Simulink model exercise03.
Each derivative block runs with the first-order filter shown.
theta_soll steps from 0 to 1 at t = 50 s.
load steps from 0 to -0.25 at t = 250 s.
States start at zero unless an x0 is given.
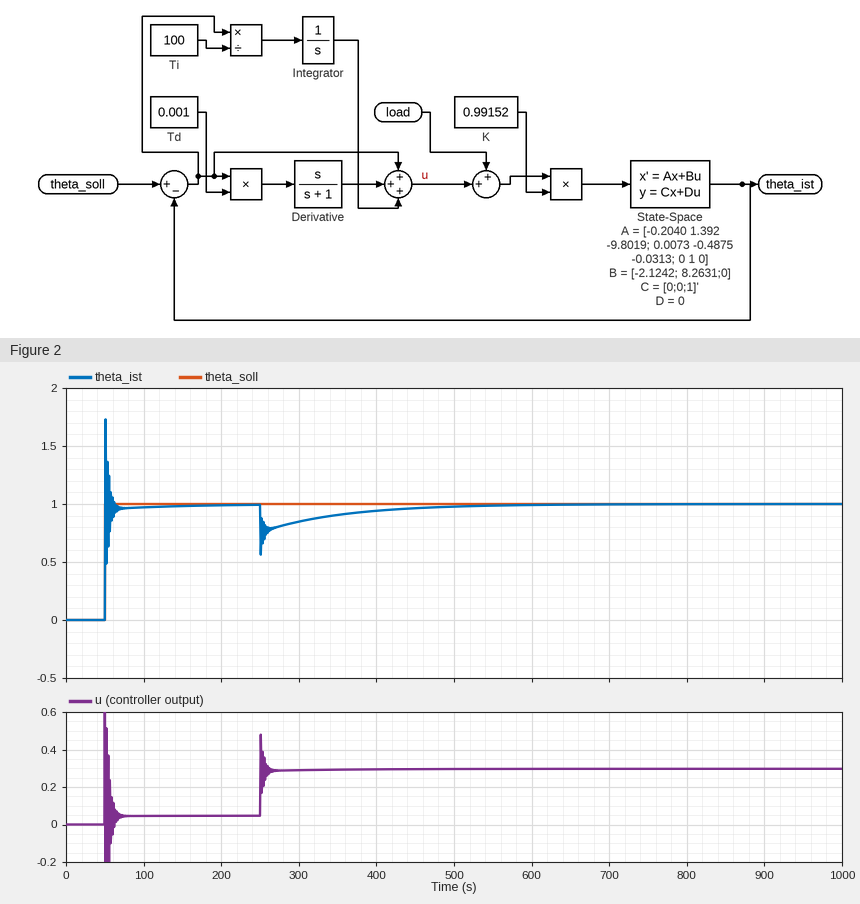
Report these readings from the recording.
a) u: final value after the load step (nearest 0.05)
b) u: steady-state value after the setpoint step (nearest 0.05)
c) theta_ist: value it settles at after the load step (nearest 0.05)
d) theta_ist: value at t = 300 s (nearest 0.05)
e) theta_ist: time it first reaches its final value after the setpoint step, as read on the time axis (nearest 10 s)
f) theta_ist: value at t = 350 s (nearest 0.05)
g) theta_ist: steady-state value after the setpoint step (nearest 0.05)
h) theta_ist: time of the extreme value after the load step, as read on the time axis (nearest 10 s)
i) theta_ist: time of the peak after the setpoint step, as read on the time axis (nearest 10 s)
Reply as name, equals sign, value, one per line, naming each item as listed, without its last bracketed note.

u: final value after the load step = 0.30
u: steady-state value after the setpoint step = 0.05
theta_ist: value it settles at after the load step = 1.00
theta_ist: value at t = 300 s = 0.85
theta_ist: time it first reaches its final value after the setpoint step, as read on the time axis = 50 s
theta_ist: value at t = 350 s = 0.90
theta_ist: steady-state value after the setpoint step = 1.00
theta_ist: time of the extreme value after the load step, as read on the time axis = 250 s
theta_ist: time of the peak after the setpoint step, as read on the time axis = 50 s
